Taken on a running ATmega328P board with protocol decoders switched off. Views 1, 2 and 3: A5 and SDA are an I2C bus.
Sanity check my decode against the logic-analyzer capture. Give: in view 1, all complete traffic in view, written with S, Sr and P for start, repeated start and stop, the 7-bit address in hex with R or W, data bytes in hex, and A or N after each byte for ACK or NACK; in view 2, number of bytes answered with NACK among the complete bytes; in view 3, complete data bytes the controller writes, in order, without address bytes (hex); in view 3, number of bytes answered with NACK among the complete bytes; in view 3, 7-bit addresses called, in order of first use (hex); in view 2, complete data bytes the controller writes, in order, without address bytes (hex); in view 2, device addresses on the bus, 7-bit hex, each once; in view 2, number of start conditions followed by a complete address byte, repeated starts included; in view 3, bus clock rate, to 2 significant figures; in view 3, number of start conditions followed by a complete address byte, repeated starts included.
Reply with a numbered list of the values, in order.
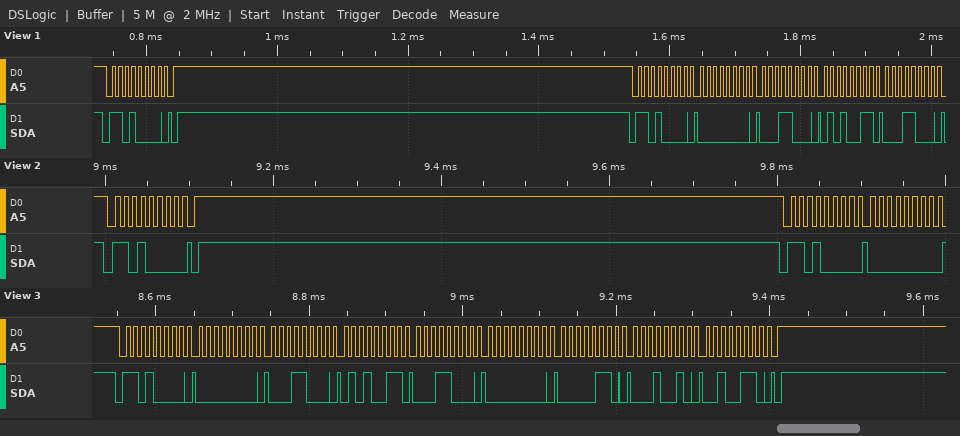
1. S 68W A P S 68W A 00 A 18 A 53 A 18 A
2. 0
3. 00 18 53 18 00 06 12 26
4. 0
5. 0x68
6. 00
7. 0x68
8. 2
9. 100 kHz
10. 1
